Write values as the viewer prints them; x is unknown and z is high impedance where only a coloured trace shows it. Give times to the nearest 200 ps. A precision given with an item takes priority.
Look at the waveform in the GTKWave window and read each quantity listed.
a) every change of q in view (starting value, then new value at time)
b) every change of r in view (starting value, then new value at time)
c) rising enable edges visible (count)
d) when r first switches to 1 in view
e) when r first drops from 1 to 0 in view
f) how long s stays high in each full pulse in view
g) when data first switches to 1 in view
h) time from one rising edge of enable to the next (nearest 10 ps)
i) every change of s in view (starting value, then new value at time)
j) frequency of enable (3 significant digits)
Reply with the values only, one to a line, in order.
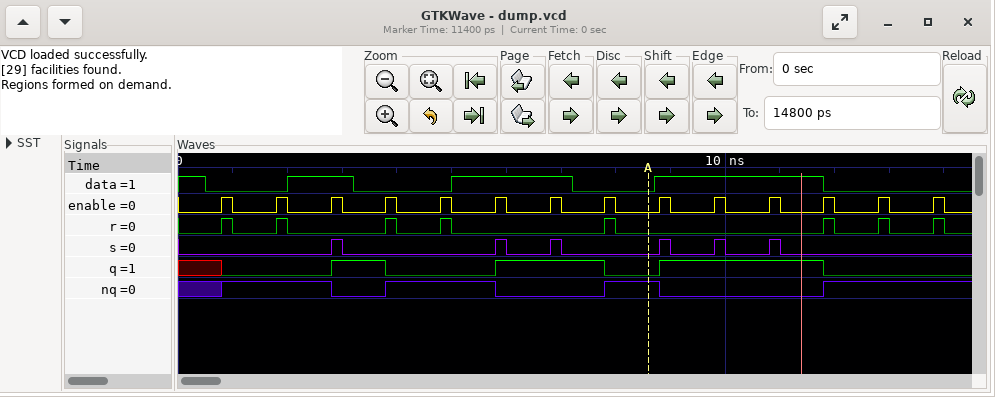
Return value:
x, 0 at 800 ps, 1 at 2800 ps, 0 at 3800 ps, 1 at 5800 ps, 0 at 7800 ps, 1 at 8800 ps, 0 at 11800 ps
0, 1 at 800 ps, 0 at 1000 ps, 1 at 1800 ps, 0 at 2000 ps, 1 at 3800 ps, 0 at 4000 ps, 1 at 4800 ps, 0 at 5000 ps, 1 at 7800 ps, 0 at 8000 ps, 1 at 11800 ps, 0 at 12000 ps, 1 at 12800 ps, 0 at 13000 ps, 1 at 13800 ps, 0 at 14000 ps
14
800 ps
1000 ps
200 ps, 200 ps, 200 ps, 200 ps, 200 ps, 200 ps
2000 ps
1000 ps
0, 1 at 2800 ps, 0 at 3000 ps, 1 at 5800 ps, 0 at 6000 ps, 1 at 6800 ps, 0 at 7000 ps, 1 at 8800 ps, 0 at 9000 ps, 1 at 9800 ps, 0 at 10000 ps, 1 at 10800 ps, 0 at 11000 ps
1.00 GHz
